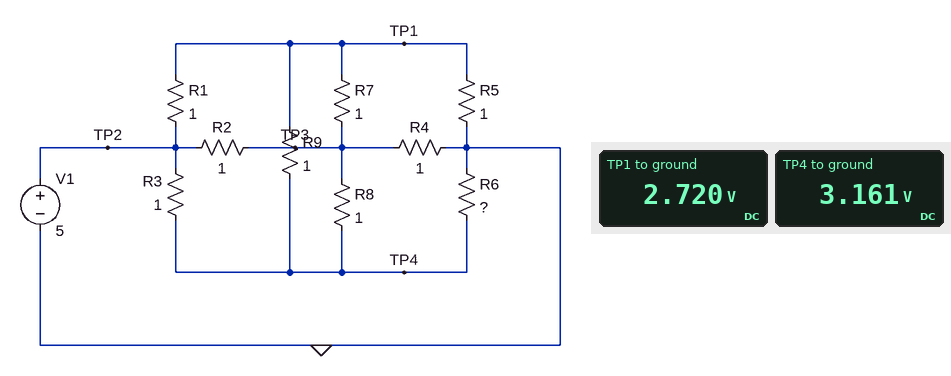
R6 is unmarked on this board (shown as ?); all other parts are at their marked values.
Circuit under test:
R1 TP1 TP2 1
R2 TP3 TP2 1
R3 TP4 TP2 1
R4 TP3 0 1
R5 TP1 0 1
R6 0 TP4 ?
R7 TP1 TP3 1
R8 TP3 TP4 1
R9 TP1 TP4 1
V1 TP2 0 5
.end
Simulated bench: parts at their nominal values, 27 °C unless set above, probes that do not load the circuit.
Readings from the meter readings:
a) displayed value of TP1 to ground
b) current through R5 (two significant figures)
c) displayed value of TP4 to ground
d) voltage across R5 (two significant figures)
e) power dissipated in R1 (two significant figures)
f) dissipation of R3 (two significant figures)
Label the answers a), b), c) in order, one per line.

a) 2.720 V
b) 2.7 A
c) 3.161 V
d) 2.7 V
e) 5.2 W
f) 3.4 W
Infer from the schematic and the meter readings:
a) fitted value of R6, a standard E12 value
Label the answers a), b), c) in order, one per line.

a) 3.3 Ω
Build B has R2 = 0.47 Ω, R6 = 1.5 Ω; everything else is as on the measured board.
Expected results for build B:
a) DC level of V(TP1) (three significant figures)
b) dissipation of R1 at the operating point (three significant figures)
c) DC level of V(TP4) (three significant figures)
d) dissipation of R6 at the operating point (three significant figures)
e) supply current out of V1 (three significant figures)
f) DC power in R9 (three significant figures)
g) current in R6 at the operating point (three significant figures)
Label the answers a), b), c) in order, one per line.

a) 2.80 V
b) 4.83 W
c) 3.00 V
d) 6.01 W
e) 8.01 A
f) 40.1 mW
g) 2.00 A
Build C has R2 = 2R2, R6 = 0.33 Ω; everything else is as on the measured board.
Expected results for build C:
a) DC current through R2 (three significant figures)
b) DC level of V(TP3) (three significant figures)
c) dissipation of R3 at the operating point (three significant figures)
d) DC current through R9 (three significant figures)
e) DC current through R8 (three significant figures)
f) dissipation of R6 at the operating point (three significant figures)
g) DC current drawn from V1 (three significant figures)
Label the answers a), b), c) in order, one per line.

a) 1.52 A
b) 1.66 V
c) 12.7 W
d) 585 mA
e) 221 mA
f) 6.29 W
g) 8.05 A
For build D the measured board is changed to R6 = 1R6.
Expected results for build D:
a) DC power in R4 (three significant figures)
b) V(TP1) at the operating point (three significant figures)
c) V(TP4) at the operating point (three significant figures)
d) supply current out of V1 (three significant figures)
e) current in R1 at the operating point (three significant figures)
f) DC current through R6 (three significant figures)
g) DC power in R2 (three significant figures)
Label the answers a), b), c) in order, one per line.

a) 6.79 W
b) 2.61 V
c) 2.82 V
d) 6.97 A
e) 2.39 A
f) 1.76 A
g) 5.73 W
